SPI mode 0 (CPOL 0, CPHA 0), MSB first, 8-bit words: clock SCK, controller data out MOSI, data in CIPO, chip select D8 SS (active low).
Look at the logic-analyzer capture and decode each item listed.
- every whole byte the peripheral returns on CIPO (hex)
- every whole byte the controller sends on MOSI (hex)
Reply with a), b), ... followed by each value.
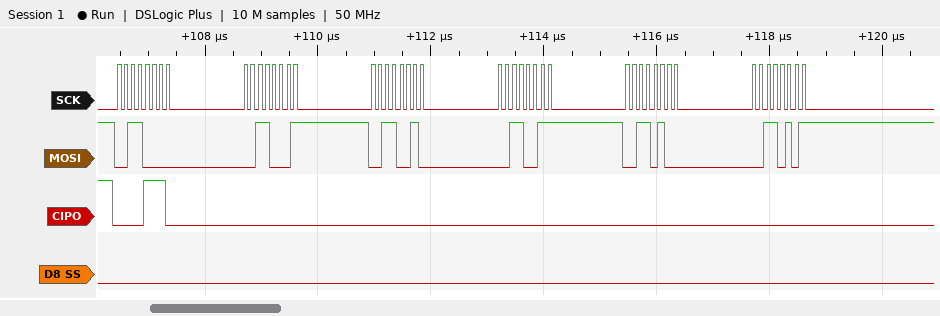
a) 0E 00 00 00 00 00
b) 30 31 32 33 34 35
